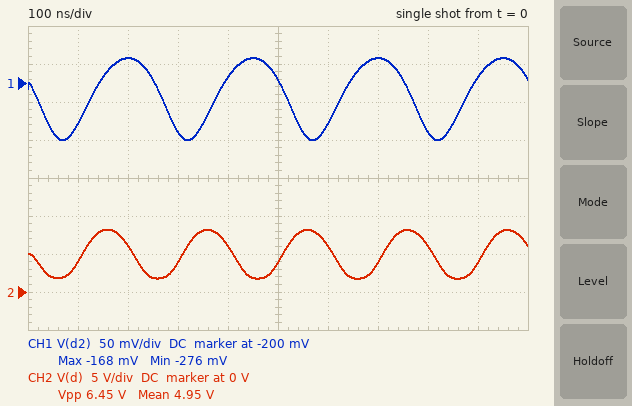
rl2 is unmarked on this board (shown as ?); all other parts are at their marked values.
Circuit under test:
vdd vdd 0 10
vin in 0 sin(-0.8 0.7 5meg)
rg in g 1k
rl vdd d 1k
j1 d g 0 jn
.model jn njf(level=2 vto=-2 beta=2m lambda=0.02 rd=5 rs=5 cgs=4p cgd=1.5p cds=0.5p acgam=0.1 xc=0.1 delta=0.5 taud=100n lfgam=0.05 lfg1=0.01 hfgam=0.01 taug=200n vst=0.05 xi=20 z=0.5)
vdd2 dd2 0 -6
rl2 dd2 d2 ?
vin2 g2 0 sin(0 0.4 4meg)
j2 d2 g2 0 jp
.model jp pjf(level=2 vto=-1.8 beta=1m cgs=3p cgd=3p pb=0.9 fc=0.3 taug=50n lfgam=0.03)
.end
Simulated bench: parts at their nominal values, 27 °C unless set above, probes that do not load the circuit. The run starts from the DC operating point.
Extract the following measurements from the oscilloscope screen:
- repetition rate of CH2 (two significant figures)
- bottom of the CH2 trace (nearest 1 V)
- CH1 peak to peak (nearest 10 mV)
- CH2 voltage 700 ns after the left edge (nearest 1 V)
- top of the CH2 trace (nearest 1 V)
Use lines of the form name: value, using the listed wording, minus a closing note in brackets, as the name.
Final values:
repetition rate of CH2: 5.0 MHz
bottom of the CH2 trace: 2 V
CH1 peak to peak: 110 mV
CH2 voltage 700 ns after the left edge: 4 V
top of the CH2 trace: 8 V
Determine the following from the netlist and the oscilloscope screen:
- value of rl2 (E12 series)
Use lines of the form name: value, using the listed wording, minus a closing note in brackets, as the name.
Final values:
value of rl2: 8.2 kΩ
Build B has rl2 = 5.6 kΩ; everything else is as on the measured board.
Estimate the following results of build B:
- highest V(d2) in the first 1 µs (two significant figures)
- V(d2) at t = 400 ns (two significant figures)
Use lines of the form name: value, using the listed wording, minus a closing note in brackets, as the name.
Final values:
highest V(d2) in the first 1 µs: -250 mV
V(d2) at t = 400 ns: -280 mV
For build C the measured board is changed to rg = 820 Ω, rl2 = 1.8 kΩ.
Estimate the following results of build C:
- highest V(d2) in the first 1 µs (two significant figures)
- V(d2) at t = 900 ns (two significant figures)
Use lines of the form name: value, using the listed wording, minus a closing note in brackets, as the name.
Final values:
highest V(d2) in the first 1 µs: -820 mV
V(d2) at t = 900 ns: -940 mV
